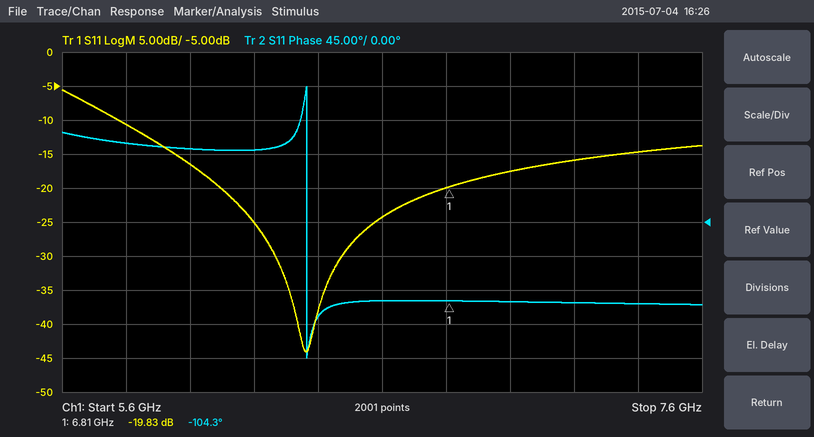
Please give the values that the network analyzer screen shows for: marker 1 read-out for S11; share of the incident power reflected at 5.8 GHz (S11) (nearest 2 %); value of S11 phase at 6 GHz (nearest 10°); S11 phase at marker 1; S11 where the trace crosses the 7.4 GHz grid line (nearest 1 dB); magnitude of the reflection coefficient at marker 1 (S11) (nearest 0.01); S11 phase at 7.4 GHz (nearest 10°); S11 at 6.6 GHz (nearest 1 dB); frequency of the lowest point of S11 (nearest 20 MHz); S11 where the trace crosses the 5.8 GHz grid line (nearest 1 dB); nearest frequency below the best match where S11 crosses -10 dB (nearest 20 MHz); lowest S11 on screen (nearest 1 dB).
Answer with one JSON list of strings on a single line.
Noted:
["-19.83 dB", "8 %", "100°", "-104.3°", "-15 dB", "0.10", "-110°", "-24 dB", "6.36 GHz", "-11 dB", "5.78 GHz", "-44 dB"]
